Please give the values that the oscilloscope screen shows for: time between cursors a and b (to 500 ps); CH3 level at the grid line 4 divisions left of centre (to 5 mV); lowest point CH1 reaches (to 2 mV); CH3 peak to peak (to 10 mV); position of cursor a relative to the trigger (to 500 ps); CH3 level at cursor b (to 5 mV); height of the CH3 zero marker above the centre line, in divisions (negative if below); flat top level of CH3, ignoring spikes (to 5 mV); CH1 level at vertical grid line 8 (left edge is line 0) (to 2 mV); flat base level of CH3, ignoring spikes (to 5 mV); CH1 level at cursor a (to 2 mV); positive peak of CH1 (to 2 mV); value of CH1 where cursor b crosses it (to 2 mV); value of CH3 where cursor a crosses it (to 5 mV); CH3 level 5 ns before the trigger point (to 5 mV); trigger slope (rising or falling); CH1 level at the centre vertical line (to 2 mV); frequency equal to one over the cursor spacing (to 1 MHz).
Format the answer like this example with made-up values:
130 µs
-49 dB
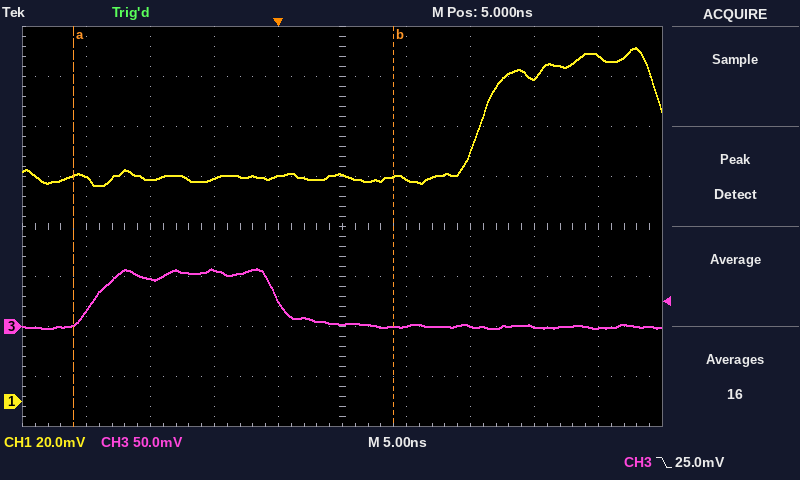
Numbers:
25.0 ns
15 mV
86 mV
60 mV
-16.0 ns
0 mV
-2.0 div
55 mV
130 mV
0 mV
90 mV
142 mV
90 mV
0 mV
55 mV
falling
90 mV
40 MHz
